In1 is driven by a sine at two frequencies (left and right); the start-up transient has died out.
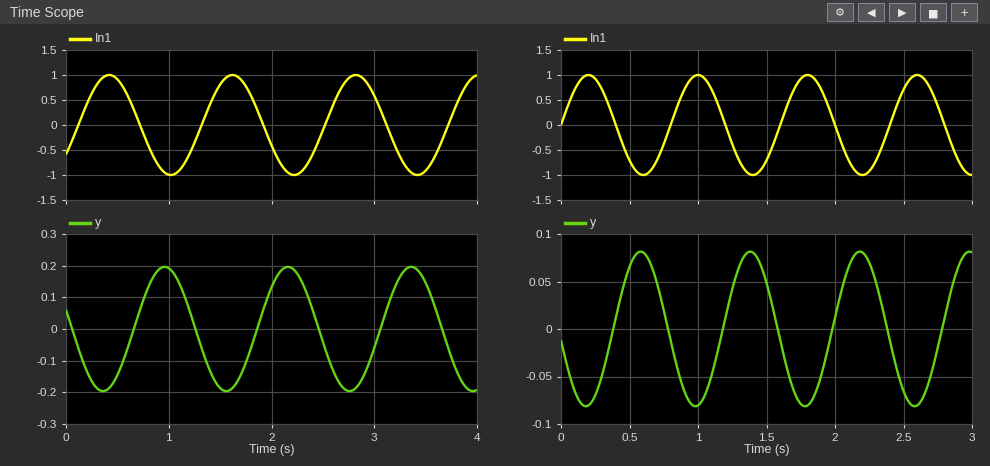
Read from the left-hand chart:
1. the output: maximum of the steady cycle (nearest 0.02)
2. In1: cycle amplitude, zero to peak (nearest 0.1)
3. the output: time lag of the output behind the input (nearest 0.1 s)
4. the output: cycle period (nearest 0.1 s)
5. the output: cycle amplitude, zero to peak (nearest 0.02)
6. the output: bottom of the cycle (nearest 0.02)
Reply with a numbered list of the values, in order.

1. 0.20
2. 1.0
3. 0.5 s
4. 1.2 s
5. 0.20
6. -0.20
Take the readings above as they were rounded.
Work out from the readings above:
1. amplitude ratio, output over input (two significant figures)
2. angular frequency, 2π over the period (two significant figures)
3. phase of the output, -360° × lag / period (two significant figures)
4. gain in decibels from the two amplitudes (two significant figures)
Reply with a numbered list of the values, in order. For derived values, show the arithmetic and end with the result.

1. 0.2 / 1 = 0.20
2. 2π / 1.2 = 5.2 rad/s
3. -360 × 0.5 / 1.2 = -150°
4. 20 log10(0.2 / 1) = -14 dB
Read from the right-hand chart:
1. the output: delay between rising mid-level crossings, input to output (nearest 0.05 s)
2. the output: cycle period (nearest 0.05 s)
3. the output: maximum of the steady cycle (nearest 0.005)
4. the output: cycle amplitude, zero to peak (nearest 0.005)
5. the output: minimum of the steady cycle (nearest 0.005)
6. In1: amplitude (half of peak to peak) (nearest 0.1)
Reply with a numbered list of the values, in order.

1. 0.40 s
2. 0.80 s
3. 0.080
4. 0.080
5. -0.080
6. 1.0
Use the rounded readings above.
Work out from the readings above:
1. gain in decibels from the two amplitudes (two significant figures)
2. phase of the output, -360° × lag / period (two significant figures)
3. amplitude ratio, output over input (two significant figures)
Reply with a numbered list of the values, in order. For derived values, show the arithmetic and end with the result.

1. 20 log10(0.08 / 1) = -22 dB
2. -360 × 0.4 / 0.8 = -180°
3. 0.08 / 1 = 0.080
